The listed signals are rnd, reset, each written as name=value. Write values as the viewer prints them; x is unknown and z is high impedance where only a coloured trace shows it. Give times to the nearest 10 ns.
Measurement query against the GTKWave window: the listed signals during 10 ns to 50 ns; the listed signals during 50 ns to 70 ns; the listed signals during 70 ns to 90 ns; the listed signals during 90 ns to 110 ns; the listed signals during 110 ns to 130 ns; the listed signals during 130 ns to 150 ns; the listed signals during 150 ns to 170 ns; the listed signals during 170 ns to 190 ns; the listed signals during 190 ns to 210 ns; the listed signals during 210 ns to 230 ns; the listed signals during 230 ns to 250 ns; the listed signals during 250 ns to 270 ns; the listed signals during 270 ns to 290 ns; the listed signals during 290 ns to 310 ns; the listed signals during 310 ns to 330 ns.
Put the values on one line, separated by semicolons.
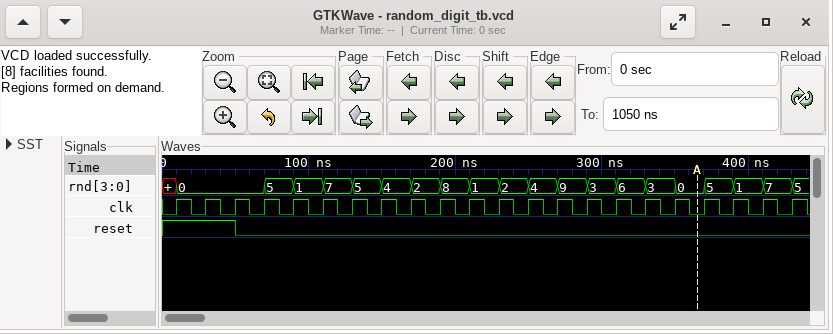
rnd=0, reset=1; rnd=0, reset=0; rnd=5, reset=0; rnd=1, reset=0; rnd=7, reset=0; rnd=5, reset=0; rnd=4, reset=0; rnd=2, reset=0; rnd=8, reset=0; rnd=1, reset=0; rnd=2, reset=0; rnd=4, reset=0; rnd=9, reset=0; rnd=3, reset=0; rnd=6, reset=0
